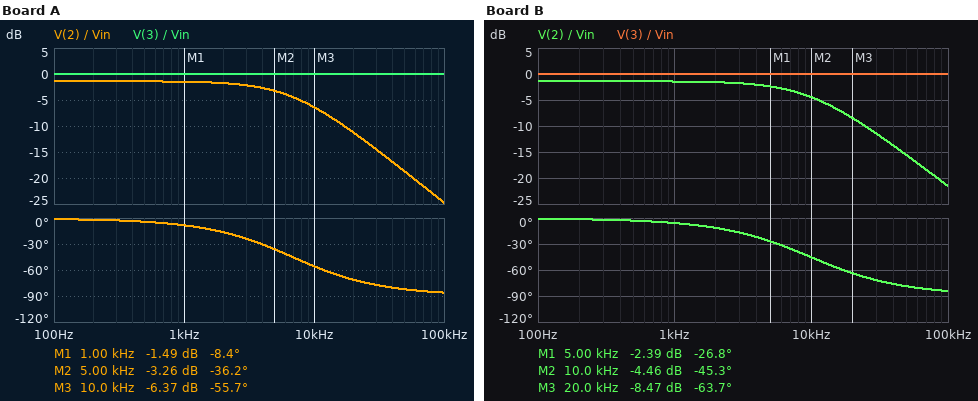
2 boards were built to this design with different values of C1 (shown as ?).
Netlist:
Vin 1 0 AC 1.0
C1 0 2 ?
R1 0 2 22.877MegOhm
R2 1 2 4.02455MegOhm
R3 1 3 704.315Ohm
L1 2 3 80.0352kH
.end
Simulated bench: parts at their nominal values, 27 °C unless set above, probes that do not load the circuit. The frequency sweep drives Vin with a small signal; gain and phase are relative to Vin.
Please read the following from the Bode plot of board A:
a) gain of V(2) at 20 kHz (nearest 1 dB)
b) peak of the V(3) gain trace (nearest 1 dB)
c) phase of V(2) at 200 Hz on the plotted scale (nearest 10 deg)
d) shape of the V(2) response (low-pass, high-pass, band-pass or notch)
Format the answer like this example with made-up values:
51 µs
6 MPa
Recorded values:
-11 dB
0 dB
0 deg
low-pass
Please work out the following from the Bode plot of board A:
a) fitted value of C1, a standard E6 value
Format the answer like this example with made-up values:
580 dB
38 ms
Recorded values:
6.8 pF
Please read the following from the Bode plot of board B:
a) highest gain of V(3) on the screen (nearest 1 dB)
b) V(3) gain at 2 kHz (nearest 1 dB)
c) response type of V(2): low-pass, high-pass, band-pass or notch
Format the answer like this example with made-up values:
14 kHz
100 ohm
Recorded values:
0 dB
0 dB
low-pass
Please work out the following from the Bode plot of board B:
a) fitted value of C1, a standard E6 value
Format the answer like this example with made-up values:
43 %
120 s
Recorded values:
4.7 pF
